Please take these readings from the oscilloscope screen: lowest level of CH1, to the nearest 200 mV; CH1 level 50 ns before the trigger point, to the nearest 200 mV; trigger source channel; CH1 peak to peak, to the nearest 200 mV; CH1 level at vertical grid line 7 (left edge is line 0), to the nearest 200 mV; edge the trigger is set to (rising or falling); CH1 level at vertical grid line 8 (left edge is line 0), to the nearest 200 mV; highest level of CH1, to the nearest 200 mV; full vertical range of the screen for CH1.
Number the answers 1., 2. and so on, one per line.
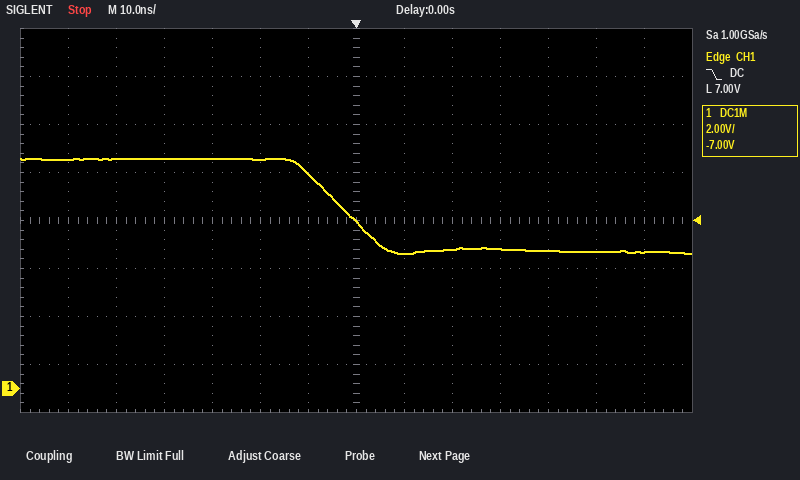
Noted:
1. 5.6 V
2. 9.6 V
3. CH1
4. 4.0 V
5. 7.0 V
6. falling
7. 5.6 V
8. 9.6 V
9. 16 V
